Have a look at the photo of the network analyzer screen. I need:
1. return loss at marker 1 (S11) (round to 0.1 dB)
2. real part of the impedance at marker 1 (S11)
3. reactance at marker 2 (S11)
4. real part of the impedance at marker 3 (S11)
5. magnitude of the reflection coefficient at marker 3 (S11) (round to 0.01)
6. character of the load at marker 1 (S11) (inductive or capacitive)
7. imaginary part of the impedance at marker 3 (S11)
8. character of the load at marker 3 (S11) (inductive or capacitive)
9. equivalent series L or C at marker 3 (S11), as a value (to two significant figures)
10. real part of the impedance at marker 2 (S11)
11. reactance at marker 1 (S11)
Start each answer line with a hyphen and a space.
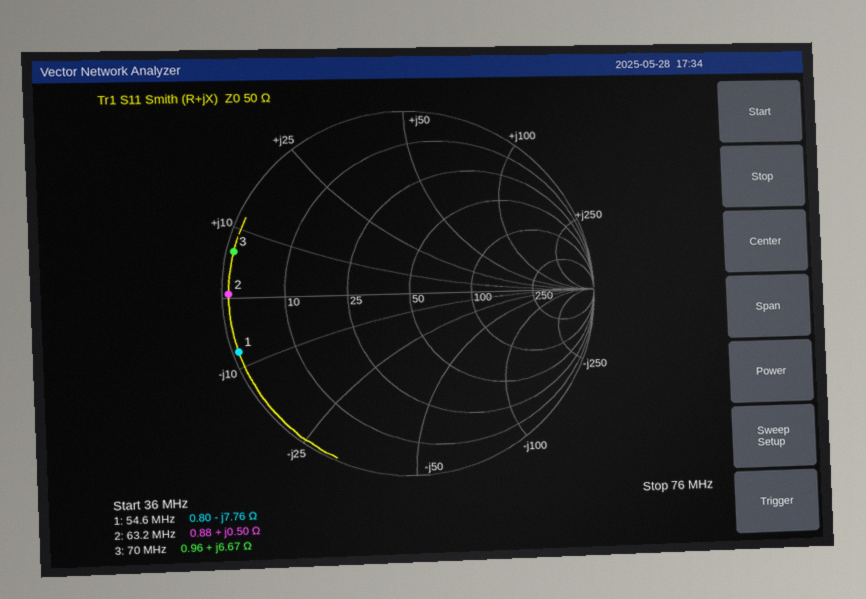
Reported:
- 0.3 dB
- 0.80 Ω
- +0.50 Ω
- 0.96 Ω
- 0.96
- capacitive
- +6.67 Ω
- inductive
- 15 nH
- 0.88 Ω
- -7.76 Ω
